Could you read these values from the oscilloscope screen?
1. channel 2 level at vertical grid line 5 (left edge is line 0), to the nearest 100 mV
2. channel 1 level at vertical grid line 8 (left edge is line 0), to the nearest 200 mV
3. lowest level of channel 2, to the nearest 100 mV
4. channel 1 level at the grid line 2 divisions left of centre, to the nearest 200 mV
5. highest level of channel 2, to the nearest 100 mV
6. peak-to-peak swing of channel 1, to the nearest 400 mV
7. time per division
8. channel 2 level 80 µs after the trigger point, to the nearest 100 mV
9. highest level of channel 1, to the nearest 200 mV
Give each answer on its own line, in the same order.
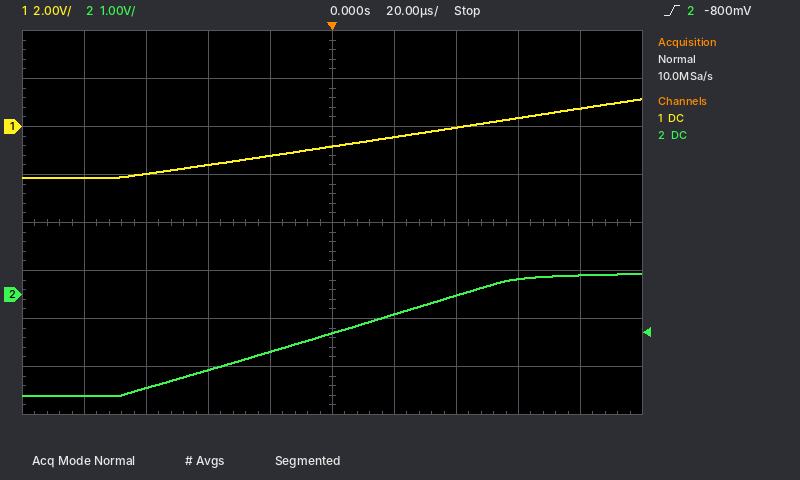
-800 mV
400 mV
-2.1 V
-1.6 V
400 mV
3.2 V
20 µs
400 mV
1.2 V
